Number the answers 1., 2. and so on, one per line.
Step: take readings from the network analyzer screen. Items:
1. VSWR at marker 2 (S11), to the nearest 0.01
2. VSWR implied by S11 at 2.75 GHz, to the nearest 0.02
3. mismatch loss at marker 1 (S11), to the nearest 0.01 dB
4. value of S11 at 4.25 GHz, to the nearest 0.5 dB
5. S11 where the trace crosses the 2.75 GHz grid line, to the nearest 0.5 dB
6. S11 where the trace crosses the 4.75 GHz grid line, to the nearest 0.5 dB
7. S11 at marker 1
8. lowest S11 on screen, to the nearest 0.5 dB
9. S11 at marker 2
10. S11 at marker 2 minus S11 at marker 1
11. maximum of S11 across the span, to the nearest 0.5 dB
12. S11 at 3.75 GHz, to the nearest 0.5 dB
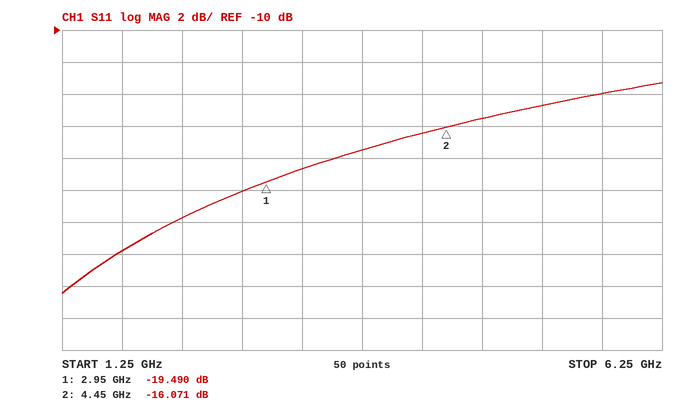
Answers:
1. 1.37
2. 1.22
3. 0.05 dB
4. -16.5 dB
5. -20.0 dB
6. -15.5 dB
7. -19.490 dB
8. -26.5 dB
9. -16.071 dB
10. 3.419 dB
11. -13.5 dB
12. -17.5 dB
